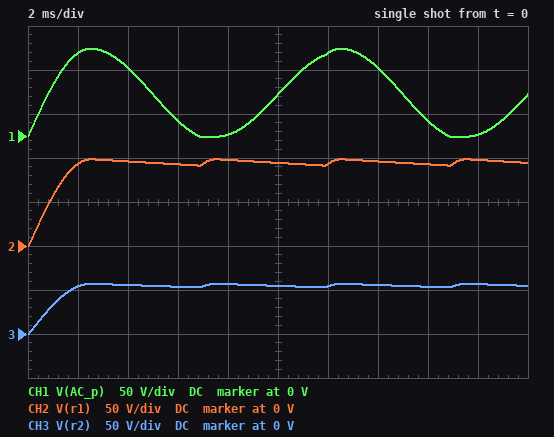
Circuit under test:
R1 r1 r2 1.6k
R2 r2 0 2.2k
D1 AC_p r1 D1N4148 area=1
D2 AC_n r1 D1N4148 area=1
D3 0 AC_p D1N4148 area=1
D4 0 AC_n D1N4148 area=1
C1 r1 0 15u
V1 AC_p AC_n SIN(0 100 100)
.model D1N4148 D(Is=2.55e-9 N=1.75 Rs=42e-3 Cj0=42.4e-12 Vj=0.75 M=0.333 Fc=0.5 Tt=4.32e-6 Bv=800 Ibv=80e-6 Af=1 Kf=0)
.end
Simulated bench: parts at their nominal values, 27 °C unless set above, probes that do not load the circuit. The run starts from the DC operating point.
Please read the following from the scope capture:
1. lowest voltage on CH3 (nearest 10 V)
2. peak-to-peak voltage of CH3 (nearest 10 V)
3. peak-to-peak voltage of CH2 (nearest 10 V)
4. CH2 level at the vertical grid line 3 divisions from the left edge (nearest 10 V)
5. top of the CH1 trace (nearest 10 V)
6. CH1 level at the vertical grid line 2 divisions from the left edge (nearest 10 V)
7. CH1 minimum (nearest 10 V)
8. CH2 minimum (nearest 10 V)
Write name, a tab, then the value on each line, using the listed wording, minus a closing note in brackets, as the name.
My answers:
lowest voltage on CH3	0 V
peak-to-peak voltage of CH3	60 V
peak-to-peak voltage of CH2	100 V
CH2 level at the vertical grid line 3 divisions from the left edge	90 V
top of the CH1 trace	100 V
CH1 level at the vertical grid line 2 divisions from the left edge	80 V
CH1 minimum	0 V
CH2 minimum	0 V
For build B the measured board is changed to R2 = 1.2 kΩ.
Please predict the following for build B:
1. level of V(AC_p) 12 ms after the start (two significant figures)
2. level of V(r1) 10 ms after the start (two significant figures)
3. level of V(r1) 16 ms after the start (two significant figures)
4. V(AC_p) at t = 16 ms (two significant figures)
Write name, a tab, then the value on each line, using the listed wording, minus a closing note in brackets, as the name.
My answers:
level of V(AC_p) 12 ms after the start	94 V
level of V(r1) 10 ms after the start	93 V
level of V(r1) 16 ms after the start	91 V
V(AC_p) at t = 16 ms	16 V
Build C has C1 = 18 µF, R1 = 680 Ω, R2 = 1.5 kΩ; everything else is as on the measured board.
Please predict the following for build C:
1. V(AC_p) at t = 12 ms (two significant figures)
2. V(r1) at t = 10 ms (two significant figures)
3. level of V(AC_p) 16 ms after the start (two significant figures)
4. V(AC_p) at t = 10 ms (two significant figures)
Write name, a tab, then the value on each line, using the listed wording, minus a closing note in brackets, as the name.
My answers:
V(AC_p) at t = 12 ms	94 V
V(r1) at t = 10 ms	93 V
level of V(AC_p) 16 ms after the start	16 V
V(AC_p) at t = 10 ms	46 V
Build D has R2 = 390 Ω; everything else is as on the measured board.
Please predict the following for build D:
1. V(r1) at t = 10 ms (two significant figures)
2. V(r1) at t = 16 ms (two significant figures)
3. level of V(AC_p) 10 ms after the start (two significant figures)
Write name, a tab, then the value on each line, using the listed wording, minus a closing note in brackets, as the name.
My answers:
V(r1) at t = 10 ms	91 V
V(r1) at t = 16 ms	88 V
level of V(AC_p) 10 ms after the start	45 V
